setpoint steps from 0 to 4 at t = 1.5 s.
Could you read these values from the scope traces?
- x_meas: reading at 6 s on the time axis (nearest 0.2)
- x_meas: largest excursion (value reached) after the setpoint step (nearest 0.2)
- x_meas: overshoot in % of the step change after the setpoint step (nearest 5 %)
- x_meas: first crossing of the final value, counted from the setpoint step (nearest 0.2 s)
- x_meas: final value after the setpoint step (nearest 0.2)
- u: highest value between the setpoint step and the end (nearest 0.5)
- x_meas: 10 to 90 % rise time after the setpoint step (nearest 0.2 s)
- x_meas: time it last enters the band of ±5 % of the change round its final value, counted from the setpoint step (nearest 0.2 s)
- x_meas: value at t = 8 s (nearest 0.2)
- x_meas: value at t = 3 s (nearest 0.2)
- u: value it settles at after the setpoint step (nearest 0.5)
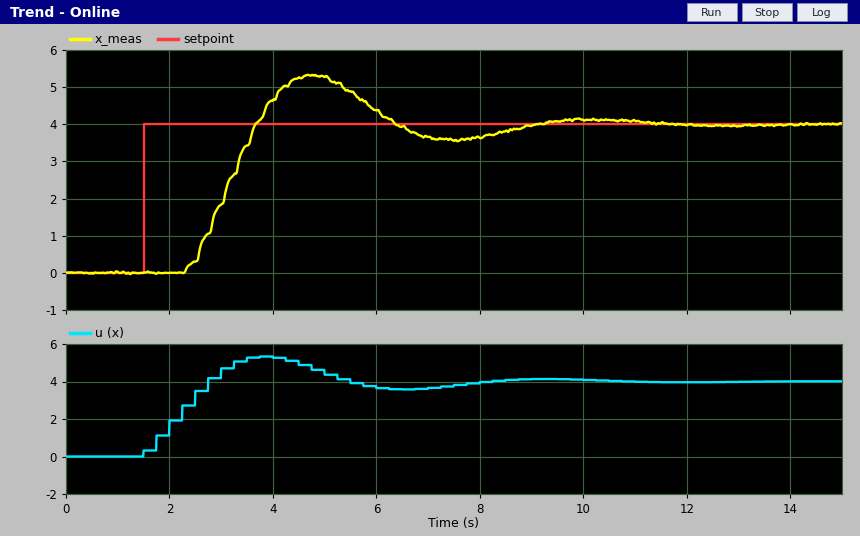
4.4
5.4
35 %
2.2 s
4.0
5.5
1.0 s
7.0 s
3.6
1.8
4.0
